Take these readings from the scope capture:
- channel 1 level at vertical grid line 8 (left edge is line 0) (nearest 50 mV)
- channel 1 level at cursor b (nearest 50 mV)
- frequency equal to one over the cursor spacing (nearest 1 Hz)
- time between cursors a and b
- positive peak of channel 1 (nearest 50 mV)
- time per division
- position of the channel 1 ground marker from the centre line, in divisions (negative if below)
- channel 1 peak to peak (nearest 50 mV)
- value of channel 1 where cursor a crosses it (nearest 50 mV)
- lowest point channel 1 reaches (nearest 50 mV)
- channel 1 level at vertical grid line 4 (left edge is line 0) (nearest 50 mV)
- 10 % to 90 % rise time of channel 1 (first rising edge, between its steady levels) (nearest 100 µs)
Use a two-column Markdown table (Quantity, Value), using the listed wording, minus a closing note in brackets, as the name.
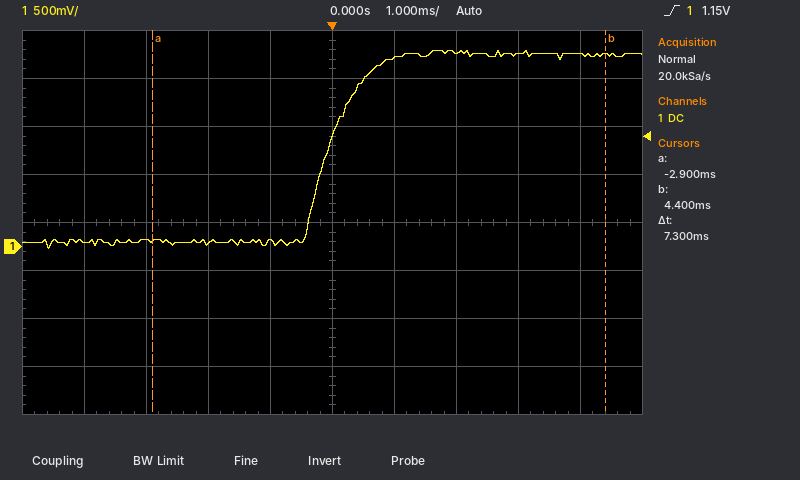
| Quantity | Value |
|---|---|
| channel 1 level at vertical grid line 8 (left edge is line 0) | 2.00 V |
| channel 1 level at cursor b | 2.00 V |
| frequency equal to one over the cursor spacing | 137 Hz |
| time between cursors a and b | 7.3 ms |
| positive peak of channel 1 | 2.05 V |
| time per division | 1 ms |
| position of the channel 1 ground marker from the centre line, in divisions | -0.5 div |
| channel 1 peak to peak | 2.05 V |
| value of channel 1 where cursor a crosses it | 50 mV |
| lowest point channel 1 reaches | 0 mV |
| channel 1 level at vertical grid line 4 (left edge is line 0) | 50 mV |
| 10 % to 90 % rise time of channel 1 (first rising edge, between its steady levels) | 1.0 ms |
